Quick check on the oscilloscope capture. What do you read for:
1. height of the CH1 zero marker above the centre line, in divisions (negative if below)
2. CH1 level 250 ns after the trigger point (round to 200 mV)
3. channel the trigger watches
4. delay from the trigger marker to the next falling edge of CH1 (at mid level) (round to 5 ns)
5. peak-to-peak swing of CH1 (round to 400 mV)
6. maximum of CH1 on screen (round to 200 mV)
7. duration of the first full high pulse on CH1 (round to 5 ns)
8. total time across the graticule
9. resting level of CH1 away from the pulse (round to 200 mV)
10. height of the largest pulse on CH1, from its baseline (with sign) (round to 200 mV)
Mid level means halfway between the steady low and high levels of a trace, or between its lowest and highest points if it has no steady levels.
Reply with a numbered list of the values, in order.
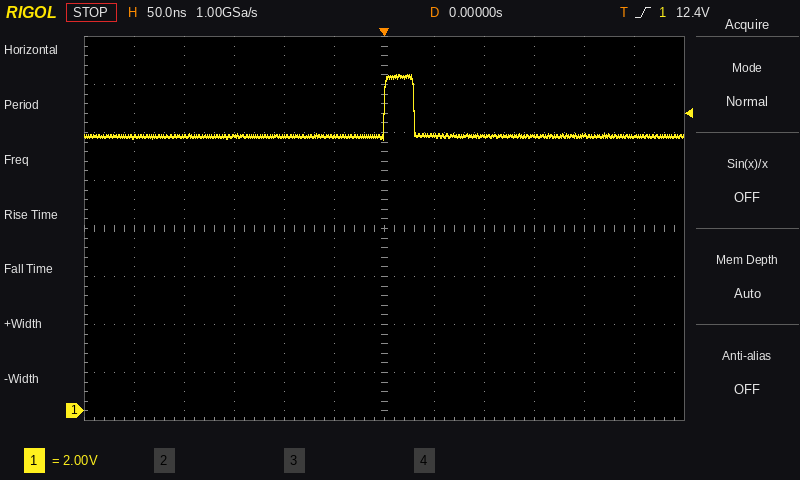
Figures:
1. -3.8 div
2. 11.4 V
3. CH1
4. 30 ns
5. 2.8 V
6. 14.0 V
7. 30 ns
8. 600 ns
9. 11.4 V
10. +2.6 V
